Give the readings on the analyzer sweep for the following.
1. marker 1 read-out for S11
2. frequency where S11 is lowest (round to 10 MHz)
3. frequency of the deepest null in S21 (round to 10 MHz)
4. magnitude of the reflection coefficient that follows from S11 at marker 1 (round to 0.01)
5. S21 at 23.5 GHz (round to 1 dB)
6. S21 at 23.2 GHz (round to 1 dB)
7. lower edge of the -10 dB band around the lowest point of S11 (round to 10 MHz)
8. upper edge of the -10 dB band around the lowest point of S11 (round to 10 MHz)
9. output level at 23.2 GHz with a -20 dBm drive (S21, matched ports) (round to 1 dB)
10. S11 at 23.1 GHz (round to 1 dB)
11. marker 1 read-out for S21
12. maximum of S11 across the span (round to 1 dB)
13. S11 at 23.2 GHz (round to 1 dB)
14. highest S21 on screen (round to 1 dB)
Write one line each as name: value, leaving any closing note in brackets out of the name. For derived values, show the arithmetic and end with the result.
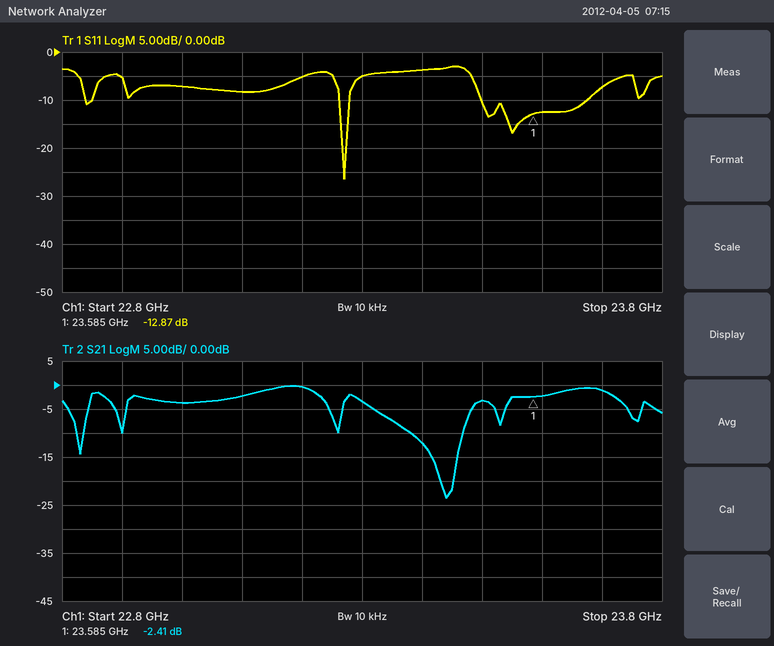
marker 1 read-out for S11: -12.87 dB
frequency where S11 is lowest: 23.27 GHz
frequency of the deepest null in S21: 23.44 GHz
magnitude of the reflection coefficient that follows from S11 at marker 1: 10^(-12.87/20) ≈ 0.23
S21 at 23.5 GHz: -3 dB
S21 at 23.2 GHz: 0 dB
lower edge of the -10 dB band around the lowest point of S11: 23.26 GHz
upper edge of the -10 dB band around the lowest point of S11: 23.28 GHz
output level at 23.2 GHz with a -20 dBm drive (S21, matched ports): -20 dBm + (0 dB) = -20 dBm
S11 at 23.1 GHz: -8 dB
marker 1 read-out for S21: -2.41 dB
maximum of S11 across the span: -3 dB
S11 at 23.2 GHz: -5 dB
highest S21 on screen: 0 dB
